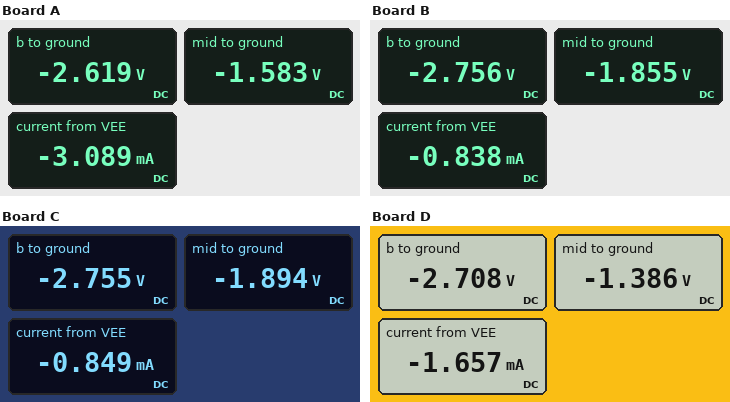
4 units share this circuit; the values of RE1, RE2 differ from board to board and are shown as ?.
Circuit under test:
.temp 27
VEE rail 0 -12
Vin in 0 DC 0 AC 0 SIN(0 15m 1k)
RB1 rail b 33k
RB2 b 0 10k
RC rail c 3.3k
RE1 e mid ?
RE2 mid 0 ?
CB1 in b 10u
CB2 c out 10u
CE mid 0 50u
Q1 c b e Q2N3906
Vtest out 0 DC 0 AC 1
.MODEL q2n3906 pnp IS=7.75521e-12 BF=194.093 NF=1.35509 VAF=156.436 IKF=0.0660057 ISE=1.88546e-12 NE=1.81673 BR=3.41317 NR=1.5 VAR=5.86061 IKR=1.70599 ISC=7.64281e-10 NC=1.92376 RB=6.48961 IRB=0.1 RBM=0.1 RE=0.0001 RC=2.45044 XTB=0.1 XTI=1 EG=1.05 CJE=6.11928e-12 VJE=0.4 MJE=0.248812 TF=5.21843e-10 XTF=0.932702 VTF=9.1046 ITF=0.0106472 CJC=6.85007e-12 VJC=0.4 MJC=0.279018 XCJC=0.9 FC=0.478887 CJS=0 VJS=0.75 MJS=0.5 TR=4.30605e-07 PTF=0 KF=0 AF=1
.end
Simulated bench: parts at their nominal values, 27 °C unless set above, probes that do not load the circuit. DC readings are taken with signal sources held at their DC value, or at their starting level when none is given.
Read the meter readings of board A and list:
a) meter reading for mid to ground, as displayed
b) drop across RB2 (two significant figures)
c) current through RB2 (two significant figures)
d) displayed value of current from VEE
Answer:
-1.583 V
2.6 V
260 µA
-3.089 mA
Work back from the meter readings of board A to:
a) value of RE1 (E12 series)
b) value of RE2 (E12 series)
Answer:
120 Ω
560 Ω
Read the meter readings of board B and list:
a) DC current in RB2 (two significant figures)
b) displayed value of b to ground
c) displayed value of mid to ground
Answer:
280 µA
-2.756 V
-1.855 V
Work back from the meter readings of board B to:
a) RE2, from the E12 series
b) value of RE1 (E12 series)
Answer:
3.3 kΩ
470 Ω
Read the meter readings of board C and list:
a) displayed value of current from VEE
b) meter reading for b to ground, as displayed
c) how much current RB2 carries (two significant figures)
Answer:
-0.849 mA
-2.755 V
280 µA
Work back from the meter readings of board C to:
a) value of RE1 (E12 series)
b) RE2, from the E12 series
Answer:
390 Ω
3.3 kΩ
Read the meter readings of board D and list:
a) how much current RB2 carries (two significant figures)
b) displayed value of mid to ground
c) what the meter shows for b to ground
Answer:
270 µA
-1.386 V
-2.708 V
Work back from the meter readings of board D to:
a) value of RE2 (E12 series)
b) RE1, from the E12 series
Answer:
1 kΩ
470 Ω
